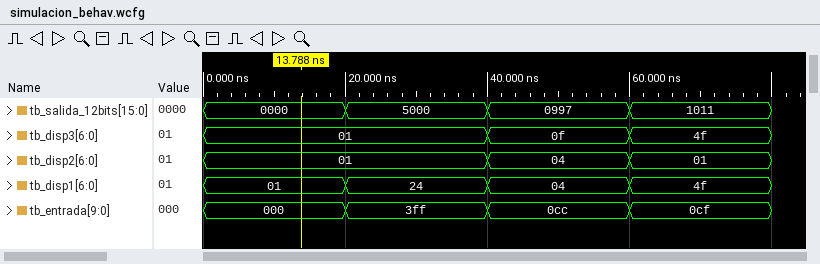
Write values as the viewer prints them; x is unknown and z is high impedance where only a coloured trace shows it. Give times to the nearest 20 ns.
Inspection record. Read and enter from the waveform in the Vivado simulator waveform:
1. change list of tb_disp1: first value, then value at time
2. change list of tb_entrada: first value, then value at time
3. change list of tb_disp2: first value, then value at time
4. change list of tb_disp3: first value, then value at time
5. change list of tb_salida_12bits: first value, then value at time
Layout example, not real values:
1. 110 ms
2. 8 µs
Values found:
1. 01, 24 at 20 ns, 04 at 40 ns, 4f at 60 ns
2. 000, 3ff at 20 ns, 0cc at 40 ns, 0cf at 60 ns
3. 01, 04 at 40 ns, 01 at 60 ns
4. 01, 0f at 40 ns, 4f at 60 ns
5. 0000, 5000 at 20 ns, 0997 at 40 ns, 1011 at 60 ns
